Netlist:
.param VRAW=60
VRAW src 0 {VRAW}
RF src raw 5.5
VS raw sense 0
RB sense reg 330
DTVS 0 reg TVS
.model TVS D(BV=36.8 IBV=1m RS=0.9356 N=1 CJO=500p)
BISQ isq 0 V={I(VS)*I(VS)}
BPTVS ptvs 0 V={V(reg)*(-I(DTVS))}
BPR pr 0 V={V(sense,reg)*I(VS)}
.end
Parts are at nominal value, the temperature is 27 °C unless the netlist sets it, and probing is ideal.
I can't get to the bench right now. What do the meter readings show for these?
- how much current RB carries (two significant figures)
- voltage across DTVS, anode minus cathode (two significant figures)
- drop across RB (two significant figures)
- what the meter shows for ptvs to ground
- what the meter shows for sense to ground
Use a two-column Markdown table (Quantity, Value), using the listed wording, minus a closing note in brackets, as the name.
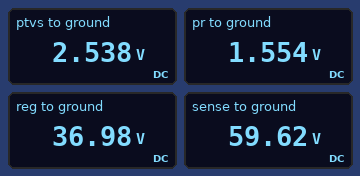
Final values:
| Quantity | Value |
|---|---|
| how much current RB carries | 69 mA |
| voltage across DTVS, anode minus cathode | -37 V |
| drop across RB | 23 V |
| what the meter shows for ptvs to ground | 2.538 V |
| what the meter shows for sense to ground | 59.62 V |
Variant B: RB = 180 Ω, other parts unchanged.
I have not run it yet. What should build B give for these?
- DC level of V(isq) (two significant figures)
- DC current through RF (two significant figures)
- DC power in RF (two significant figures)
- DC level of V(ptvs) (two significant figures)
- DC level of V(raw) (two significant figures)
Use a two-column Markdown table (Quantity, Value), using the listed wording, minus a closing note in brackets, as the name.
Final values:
| Quantity | Value |
|---|---|
| DC level of V(isq) | 15 mV |
| DC current through RF | 120 mA |
| DC power in RF | 84 mW |
| DC level of V(ptvs) | 4.6 V |
| DC level of V(raw) | 59 V |
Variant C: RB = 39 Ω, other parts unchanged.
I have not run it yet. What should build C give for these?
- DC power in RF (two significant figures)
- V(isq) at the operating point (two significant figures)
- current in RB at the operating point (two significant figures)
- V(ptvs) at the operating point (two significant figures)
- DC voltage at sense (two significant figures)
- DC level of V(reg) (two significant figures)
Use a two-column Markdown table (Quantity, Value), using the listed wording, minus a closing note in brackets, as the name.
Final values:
| Quantity | Value |
|---|---|
| DC power in RF | 1.4 W |
| V(isq) at the operating point | 260 mV |
| current in RB at the operating point | 510 mA |
| V(ptvs) at the operating point | 19 V |
| DC voltage at sense | 57 V |
| DC level of V(reg) | 37 V |
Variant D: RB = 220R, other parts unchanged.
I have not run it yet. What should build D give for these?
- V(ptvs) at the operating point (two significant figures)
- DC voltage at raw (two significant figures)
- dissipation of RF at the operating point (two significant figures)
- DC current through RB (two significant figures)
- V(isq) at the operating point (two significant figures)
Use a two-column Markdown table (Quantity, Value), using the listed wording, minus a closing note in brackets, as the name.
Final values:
| Quantity | Value |
|---|---|
| V(ptvs) at the operating point | 3.8 V |
| DC voltage at raw | 59 V |
| dissipation of RF at the operating point | 57 mW |
| DC current through RB | 100 mA |
| V(isq) at the operating point | 10 mV |
